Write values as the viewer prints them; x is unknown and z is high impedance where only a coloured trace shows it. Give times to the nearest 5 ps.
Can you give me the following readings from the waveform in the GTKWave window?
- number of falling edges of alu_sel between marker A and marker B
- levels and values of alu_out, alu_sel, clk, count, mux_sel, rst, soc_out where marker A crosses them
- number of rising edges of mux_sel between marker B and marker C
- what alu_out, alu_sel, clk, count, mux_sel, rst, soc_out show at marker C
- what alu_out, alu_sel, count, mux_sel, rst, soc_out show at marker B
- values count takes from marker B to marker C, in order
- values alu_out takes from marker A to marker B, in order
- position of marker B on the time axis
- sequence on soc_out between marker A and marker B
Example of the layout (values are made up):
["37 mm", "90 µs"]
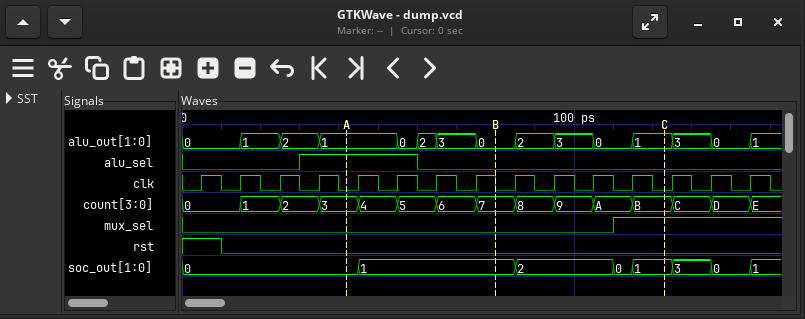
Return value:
["1", "alu_out=1, alu_sel=1, clk=0, count=3, mux_sel=0, rst=0, soc_out=0", "1", "alu_out=1, alu_sel=0, clk=0, count=B, mux_sel=1, rst=0, soc_out=1", "alu_out=0, alu_sel=0, count=7, mux_sel=0, rst=0, soc_out=1", "7, 8, 9, A, B", "1, 0, 2, 3, 0", "80 ps", "0, 1"]
